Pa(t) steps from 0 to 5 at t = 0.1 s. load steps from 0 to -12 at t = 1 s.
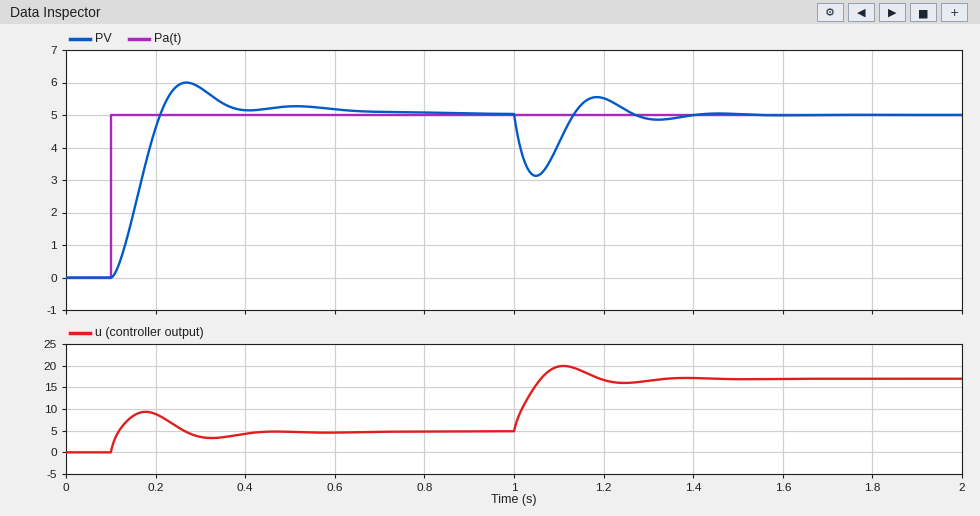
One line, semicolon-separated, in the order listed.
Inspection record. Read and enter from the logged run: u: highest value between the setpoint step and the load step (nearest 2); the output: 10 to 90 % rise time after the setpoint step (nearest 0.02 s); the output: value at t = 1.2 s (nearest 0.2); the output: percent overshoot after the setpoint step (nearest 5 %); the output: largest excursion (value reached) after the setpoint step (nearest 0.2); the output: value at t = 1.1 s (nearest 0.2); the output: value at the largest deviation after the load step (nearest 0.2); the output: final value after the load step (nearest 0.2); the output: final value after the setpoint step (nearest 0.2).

10; 0.08 s; 5.6; 20 %; 6.0; 4.2; 3.2; 5.0; 5.0
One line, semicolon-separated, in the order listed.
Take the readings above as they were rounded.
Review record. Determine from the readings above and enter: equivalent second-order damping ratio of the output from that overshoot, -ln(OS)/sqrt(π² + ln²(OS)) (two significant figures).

0.46
